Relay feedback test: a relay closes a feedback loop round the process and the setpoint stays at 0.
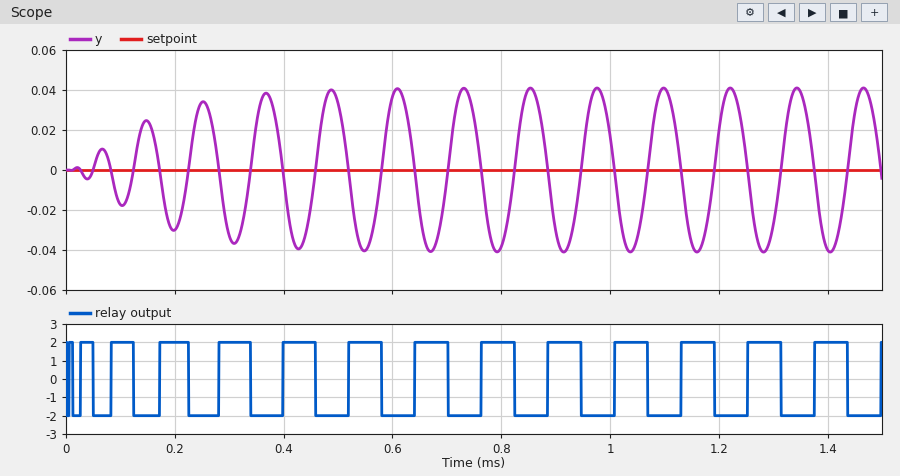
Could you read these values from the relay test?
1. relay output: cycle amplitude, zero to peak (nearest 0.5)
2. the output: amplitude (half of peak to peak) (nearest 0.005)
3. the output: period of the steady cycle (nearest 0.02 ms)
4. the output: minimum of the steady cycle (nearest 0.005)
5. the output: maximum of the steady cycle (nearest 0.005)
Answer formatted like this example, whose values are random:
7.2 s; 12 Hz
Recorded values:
2.0; 0.040; 0.12 ms; -0.040; 0.040
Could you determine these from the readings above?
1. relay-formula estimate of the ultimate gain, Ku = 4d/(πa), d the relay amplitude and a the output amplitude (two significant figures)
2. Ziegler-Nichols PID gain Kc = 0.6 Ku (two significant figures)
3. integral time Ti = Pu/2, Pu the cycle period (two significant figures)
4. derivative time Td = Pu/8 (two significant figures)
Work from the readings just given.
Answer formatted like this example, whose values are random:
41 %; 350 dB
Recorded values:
64; 38; 0.060 ms; 0.015 ms
